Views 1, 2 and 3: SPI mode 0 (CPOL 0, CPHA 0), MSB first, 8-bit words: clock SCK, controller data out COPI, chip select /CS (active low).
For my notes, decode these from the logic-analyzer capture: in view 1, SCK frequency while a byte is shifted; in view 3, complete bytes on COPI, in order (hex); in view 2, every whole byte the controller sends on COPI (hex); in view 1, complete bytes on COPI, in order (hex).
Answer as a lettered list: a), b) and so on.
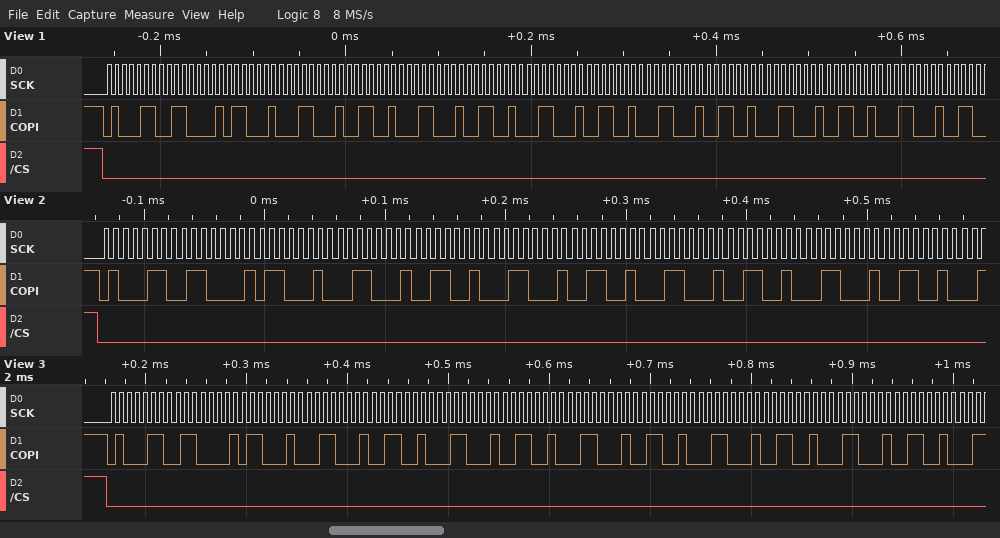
a) 125 kHz
b) 46 61 62 31 32 31 32 31 32 31 32 31 32
c) 0x46 0x61 0x62 0x31 0x32 0x31 0x32 0x31 0x32 0x31 0x32
d) 46 61 62 31 32 31 32 31 32 31 32 31 32 31
